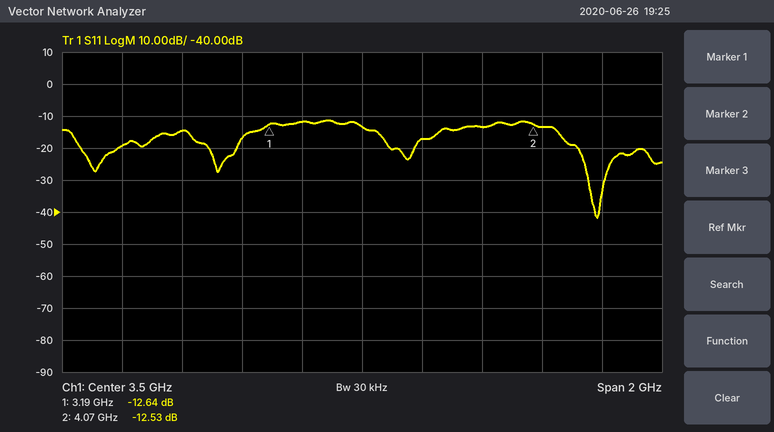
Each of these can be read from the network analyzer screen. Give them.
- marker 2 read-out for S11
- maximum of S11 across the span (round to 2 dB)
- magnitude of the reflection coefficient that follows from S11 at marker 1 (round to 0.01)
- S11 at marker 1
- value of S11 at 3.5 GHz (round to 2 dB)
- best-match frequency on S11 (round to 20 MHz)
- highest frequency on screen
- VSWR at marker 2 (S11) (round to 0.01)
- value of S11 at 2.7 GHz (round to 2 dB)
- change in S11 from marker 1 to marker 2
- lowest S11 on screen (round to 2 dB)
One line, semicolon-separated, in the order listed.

-12.53 dB; -12 dB; 0.23; -12.64 dB; -14 dB; 4.28 GHz; 4.5 GHz; 1.62; -20 dB; 0.11 dB; -42 dB
